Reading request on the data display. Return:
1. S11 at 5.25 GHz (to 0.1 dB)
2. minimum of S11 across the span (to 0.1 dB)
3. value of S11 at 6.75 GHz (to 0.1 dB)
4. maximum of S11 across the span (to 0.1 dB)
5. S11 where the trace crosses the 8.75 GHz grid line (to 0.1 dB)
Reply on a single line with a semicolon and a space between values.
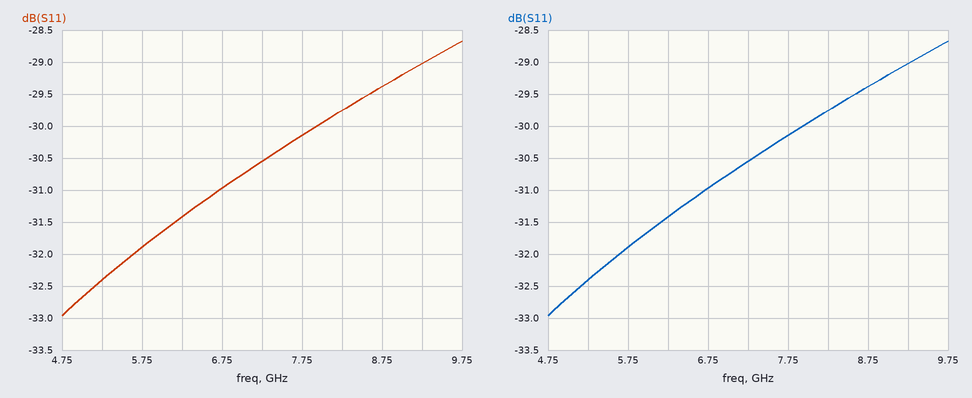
-32.4 dB; -33.0 dB; -31.0 dB; -28.7 dB; -29.4 dB
